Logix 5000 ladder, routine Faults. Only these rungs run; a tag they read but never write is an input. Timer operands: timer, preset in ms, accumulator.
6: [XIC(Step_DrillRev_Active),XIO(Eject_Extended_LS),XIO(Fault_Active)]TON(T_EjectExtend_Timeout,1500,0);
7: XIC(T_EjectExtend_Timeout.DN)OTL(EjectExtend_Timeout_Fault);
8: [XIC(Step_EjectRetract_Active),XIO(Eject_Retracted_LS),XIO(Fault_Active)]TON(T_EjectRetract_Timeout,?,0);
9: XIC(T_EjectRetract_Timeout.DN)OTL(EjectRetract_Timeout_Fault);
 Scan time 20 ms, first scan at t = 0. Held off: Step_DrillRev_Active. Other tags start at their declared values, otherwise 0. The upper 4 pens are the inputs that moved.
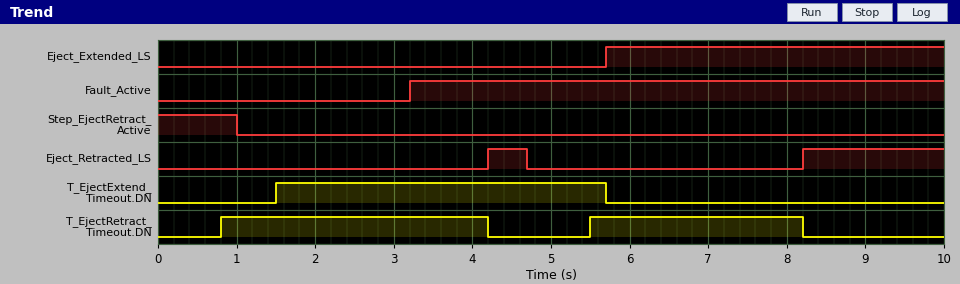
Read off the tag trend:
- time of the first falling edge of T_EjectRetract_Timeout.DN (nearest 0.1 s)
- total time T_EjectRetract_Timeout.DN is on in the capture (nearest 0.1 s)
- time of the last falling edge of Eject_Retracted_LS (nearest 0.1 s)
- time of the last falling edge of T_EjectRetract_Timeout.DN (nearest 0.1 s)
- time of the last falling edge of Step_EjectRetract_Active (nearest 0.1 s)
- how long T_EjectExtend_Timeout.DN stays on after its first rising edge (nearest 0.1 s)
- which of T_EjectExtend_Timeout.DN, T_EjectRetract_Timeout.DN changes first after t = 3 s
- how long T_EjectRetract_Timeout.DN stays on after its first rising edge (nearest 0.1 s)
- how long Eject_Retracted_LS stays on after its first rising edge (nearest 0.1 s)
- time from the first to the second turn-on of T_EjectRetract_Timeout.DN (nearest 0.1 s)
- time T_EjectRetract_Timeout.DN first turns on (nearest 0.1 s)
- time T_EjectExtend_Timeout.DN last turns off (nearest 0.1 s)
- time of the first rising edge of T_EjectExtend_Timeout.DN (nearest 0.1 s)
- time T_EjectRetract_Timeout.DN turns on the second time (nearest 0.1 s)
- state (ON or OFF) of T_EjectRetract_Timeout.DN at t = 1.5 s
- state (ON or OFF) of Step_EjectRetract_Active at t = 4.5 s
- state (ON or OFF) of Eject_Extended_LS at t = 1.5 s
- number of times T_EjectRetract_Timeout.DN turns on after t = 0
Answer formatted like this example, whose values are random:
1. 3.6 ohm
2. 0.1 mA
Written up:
1. 4.2 s
2. 6.1 s
3. 4.7 s
4. 8.2 s
5. 1.0 s
6. 4.2 s
7. T_EjectRetract_Timeout.DN
8. 3.4 s
9. 0.5 s
10. 4.7 s
11. 0.8 s
12. 5.7 s
13. 1.5 s
14. 5.5 s
15. ON
16. OFF
17. OFF
18. 2
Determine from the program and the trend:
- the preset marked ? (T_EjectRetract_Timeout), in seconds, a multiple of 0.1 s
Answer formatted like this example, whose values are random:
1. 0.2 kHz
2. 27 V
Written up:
1. 0.8 s
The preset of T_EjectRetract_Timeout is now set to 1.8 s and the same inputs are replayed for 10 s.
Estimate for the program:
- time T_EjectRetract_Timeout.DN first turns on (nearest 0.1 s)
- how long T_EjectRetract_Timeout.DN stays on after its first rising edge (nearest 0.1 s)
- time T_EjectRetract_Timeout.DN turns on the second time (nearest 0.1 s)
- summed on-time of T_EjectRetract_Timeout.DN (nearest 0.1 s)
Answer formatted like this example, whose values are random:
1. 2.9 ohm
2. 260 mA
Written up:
1. 1.8 s
2. 2.4 s
3. 6.5 s
4. 4.1 s
